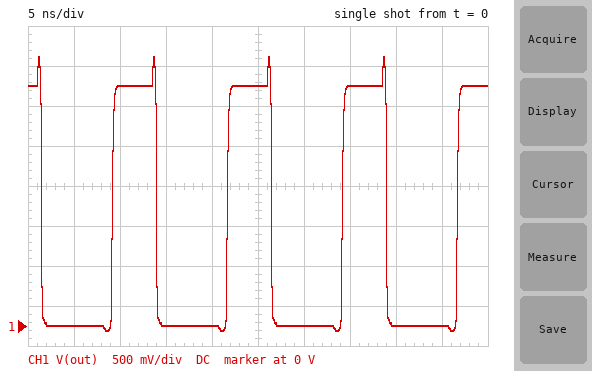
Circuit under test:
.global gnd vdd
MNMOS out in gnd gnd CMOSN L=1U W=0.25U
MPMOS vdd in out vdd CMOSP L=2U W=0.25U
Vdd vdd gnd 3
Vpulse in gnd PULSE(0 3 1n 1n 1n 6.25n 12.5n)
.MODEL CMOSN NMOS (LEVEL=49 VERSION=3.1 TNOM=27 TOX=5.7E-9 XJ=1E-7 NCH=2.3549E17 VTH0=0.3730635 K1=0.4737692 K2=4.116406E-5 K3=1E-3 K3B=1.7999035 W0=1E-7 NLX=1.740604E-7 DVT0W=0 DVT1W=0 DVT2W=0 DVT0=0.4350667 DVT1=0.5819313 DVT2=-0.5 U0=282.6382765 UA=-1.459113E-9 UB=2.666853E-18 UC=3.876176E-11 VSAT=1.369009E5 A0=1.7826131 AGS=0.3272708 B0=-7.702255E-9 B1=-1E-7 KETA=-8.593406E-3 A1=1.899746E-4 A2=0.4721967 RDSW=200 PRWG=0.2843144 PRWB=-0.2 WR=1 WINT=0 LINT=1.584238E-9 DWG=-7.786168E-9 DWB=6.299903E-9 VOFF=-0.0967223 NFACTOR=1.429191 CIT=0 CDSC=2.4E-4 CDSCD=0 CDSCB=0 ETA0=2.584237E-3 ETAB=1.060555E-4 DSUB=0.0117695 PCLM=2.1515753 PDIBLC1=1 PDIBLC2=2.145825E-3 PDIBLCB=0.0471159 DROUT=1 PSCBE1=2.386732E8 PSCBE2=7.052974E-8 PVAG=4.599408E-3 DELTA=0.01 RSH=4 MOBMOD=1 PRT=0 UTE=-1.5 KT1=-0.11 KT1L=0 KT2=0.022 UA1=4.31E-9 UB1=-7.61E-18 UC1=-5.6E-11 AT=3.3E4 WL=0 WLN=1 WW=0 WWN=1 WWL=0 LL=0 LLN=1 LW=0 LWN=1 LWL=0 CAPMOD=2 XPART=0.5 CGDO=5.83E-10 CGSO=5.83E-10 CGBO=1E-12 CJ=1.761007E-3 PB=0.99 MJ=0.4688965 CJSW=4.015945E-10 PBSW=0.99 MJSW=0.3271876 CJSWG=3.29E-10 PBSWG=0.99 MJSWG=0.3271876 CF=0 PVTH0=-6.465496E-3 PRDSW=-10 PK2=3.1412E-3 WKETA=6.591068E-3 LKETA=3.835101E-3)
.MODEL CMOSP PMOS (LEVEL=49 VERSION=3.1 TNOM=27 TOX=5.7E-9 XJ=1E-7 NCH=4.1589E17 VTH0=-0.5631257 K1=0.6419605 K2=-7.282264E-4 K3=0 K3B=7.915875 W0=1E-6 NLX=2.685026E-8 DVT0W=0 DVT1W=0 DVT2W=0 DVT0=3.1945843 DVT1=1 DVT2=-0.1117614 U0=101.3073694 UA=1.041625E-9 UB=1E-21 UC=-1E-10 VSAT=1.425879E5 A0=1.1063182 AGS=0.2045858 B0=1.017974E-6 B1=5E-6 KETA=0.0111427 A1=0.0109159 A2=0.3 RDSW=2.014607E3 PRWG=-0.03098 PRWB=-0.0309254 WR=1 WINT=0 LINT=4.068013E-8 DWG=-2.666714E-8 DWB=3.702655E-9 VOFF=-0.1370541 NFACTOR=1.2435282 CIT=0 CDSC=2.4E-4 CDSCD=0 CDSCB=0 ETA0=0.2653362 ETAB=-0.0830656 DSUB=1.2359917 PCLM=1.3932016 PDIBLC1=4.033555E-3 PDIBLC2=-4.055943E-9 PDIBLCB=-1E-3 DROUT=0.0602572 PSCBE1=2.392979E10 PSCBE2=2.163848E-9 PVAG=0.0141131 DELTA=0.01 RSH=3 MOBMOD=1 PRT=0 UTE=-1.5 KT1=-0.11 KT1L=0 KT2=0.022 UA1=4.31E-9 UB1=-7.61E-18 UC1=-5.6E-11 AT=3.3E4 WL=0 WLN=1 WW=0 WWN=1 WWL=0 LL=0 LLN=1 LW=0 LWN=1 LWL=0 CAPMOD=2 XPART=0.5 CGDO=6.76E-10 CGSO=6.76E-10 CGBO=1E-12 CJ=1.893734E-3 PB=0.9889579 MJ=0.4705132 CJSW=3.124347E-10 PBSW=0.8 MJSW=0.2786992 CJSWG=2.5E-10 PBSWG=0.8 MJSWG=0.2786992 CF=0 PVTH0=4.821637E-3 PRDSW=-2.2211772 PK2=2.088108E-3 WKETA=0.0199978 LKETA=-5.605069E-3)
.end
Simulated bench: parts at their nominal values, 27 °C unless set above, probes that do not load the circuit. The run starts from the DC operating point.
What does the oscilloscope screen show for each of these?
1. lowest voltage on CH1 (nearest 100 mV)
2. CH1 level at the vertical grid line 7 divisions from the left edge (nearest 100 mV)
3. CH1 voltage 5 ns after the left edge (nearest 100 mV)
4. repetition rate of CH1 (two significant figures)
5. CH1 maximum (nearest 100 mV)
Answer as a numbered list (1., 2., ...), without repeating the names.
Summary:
1. -100 mV
2. 3.0 V
3. 0 V
4. 80 MHz
5. 3.4 V
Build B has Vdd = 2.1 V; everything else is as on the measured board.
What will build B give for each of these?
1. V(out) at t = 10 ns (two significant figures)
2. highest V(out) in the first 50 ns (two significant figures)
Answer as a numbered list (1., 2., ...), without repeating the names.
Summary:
1. 2.1 V
2. 2.6 V
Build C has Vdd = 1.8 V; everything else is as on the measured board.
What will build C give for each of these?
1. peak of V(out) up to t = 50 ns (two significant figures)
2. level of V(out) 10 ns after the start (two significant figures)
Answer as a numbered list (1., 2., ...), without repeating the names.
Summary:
1. 2.4 V
2. 1.8 V
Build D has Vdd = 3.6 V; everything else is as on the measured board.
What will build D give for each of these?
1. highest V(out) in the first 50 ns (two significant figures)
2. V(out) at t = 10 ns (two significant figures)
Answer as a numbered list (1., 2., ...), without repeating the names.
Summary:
1. 3.9 V
2. 3.6 V
